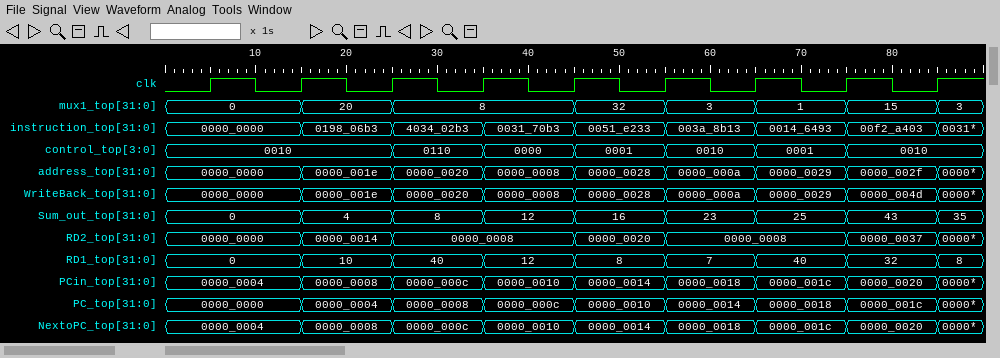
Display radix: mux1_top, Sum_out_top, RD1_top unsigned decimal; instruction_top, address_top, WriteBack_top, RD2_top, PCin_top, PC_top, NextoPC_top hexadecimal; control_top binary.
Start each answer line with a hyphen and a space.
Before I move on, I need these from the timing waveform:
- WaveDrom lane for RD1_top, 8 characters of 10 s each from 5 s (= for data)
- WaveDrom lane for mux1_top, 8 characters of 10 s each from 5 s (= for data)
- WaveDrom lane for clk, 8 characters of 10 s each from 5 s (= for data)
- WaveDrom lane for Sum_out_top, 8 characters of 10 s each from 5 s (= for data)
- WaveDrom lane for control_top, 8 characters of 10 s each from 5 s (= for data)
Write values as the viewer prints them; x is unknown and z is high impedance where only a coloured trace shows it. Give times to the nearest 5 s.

- {name: 'RD1_top', wave: '========', data: '0 10 40 12 8 7 40 32'}
- {name: 'mux1_top', wave: '===.====', data: '0 20 8 32 3 1 15'}
- {name: 'clk', wave: 'p.......'}
- {name: 'Sum_out_top', wave: '========', data: '0 4 8 12 16 23 25 43'}
- {name: 'control_top', wave: '=.======', data: '0010 0110 0000 0001 0010 0001 0010'}
